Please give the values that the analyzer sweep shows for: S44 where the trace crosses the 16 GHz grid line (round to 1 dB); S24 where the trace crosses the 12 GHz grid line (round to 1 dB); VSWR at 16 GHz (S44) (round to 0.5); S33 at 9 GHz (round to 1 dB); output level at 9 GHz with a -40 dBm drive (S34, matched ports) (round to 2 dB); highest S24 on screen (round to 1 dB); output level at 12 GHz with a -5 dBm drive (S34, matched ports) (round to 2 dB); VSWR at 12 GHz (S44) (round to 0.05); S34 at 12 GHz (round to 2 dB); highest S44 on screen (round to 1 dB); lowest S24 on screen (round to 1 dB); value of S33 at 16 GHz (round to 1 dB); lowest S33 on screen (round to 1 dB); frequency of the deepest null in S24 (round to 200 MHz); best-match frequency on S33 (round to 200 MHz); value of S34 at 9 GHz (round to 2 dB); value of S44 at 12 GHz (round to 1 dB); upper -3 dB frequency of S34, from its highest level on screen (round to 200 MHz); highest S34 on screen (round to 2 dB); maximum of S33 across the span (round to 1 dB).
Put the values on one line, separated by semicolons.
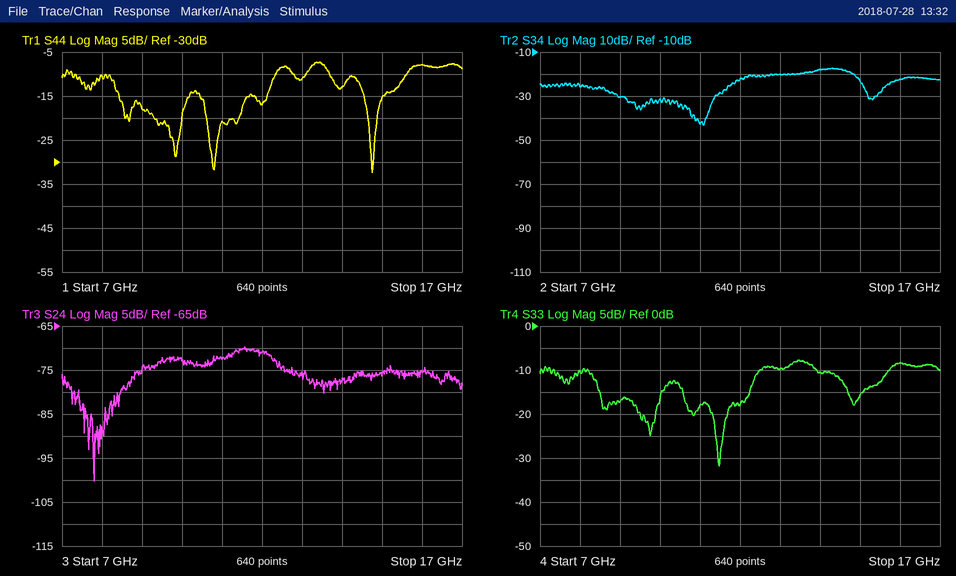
-8 dB; -71 dB; 2.5; -17 dB; -70 dBm; -70 dB; -28 dBm; 1.35; -22 dB; -7 dB; -100 dB; -8 dB; -32 dB; 7.8 GHz; 11.4 GHz; -30 dB; -17 dB; 14.8 GHz; -18 dB; -8 dB
